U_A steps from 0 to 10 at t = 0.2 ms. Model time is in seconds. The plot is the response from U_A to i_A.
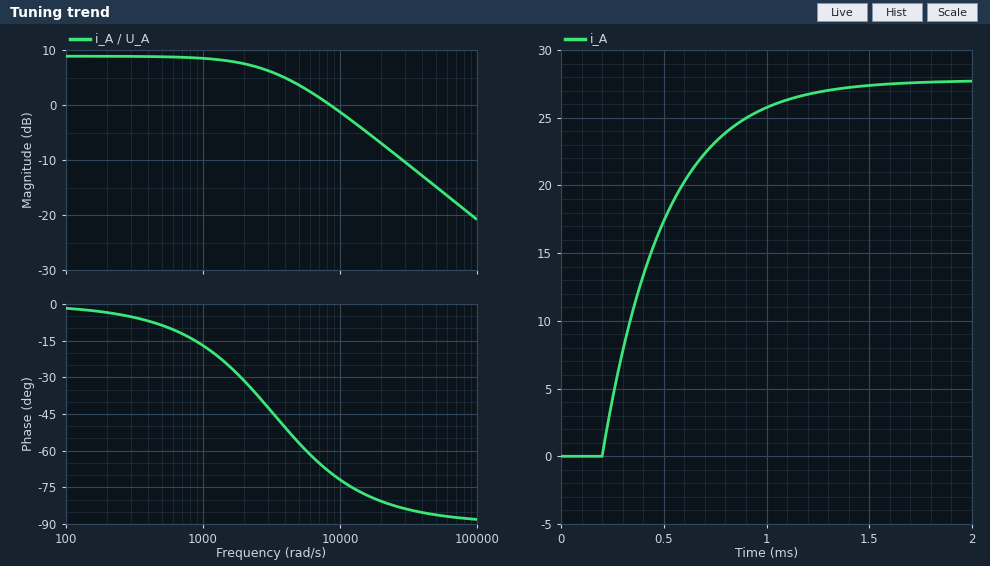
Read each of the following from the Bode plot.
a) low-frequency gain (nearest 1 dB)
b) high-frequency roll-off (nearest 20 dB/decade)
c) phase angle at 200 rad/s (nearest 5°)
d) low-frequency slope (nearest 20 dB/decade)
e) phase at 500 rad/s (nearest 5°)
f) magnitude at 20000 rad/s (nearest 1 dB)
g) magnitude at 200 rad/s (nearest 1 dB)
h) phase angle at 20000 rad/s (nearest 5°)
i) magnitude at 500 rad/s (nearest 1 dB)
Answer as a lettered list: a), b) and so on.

a) 9 dB
b) -20 dB/decade
c) -5°
d) 0 dB/decade
e) -10°
f) -7 dB
g) 9 dB
h) -80°
i) 9 dB
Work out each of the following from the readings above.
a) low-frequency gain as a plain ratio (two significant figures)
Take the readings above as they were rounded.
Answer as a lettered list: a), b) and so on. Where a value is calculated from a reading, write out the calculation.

a) 10^(9 / 20) = 2.8
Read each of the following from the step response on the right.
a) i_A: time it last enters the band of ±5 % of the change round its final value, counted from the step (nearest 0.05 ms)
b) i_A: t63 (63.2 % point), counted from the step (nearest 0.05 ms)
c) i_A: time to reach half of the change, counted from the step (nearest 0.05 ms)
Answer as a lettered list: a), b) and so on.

a) 0.90 ms
b) 0.30 ms
c) 0.20 ms
